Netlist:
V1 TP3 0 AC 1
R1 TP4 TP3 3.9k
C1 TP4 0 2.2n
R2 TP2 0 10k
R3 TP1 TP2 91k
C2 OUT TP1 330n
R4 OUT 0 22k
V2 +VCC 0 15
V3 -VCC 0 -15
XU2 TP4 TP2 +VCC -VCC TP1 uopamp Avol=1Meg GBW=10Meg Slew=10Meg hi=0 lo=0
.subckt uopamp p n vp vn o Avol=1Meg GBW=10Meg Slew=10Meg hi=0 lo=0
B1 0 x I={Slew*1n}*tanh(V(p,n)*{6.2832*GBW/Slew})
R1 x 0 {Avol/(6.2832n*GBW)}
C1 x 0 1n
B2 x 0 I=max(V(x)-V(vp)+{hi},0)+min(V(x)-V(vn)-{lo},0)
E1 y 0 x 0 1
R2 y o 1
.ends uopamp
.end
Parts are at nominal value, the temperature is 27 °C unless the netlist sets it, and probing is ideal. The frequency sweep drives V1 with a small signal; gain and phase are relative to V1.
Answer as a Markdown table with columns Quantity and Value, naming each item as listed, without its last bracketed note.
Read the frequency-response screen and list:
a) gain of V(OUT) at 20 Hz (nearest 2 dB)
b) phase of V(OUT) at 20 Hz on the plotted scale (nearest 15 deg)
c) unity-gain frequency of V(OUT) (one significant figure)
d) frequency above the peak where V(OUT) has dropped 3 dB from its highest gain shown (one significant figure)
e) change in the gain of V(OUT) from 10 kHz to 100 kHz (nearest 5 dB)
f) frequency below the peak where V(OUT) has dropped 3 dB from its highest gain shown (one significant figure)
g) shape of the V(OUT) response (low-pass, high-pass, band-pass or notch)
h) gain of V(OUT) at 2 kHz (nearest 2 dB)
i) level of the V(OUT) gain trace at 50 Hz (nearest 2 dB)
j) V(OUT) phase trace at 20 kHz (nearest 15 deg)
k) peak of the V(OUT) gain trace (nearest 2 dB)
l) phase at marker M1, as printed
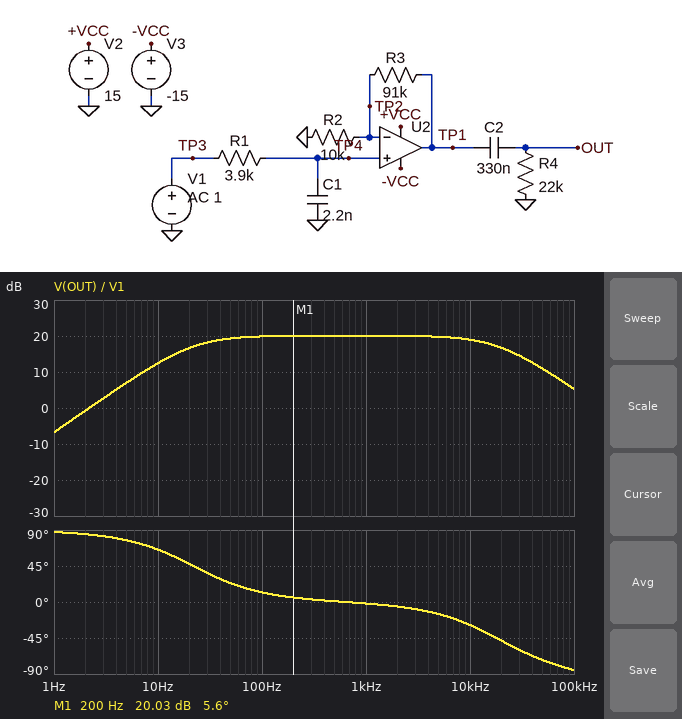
| Quantity | Value |
|---|---|
| gain of V(OUT) at 20 Hz | 16 dB |
| phase of V(OUT) at 20 Hz on the plotted scale | 45 deg |
| unity-gain frequency of V(OUT) | 2 Hz |
| frequency above the peak where V(OUT) has dropped 3 dB from its highest gain shown | 20 kHz |
| change in the gain of V(OUT) from 10 kHz to 100 kHz | -15 dB |
| frequency below the peak where V(OUT) has dropped 3 dB from its highest gain shown | 20 Hz |
| shape of the V(OUT) response | band-pass |
| gain of V(OUT) at 2 kHz | 20 dB |
| level of the V(OUT) gain trace at 50 Hz | 20 dB |
| V(OUT) phase trace at 20 kHz | -45 deg |
| peak of the V(OUT) gain trace | 20 dB |
| phase at marker M1, as printed | 5.6 deg |
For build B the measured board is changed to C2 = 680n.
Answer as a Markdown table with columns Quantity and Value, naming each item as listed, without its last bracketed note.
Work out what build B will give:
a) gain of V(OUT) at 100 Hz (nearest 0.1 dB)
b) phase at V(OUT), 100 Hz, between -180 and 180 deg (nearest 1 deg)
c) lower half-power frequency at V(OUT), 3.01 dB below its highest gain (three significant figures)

| Quantity | Value |
|---|---|
| gain of V(OUT) at 100 Hz | 20.0 dB |
| phase at V(OUT), 100 Hz, between -180 and 180 deg | 6 deg |
| lower half-power frequency at V(OUT), 3.01 dB below its highest gain | 10.6 Hz |
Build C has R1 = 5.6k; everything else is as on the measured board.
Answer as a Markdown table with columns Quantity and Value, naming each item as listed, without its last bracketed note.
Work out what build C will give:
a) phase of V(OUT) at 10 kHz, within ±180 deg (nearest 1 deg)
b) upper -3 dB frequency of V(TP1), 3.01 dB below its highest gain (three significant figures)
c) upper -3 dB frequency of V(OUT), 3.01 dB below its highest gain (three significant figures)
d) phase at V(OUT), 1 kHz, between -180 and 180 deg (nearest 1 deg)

| Quantity | Value |
|---|---|
| phase of V(OUT) at 10 kHz, within ±180 deg | -38 deg |
| upper -3 dB frequency of V(TP1), 3.01 dB below its highest gain | 12.9 kHz |
| upper -3 dB frequency of V(OUT), 3.01 dB below its highest gain | 13.0 kHz |
| phase at V(OUT), 1 kHz, between -180 and 180 deg | -3 deg |
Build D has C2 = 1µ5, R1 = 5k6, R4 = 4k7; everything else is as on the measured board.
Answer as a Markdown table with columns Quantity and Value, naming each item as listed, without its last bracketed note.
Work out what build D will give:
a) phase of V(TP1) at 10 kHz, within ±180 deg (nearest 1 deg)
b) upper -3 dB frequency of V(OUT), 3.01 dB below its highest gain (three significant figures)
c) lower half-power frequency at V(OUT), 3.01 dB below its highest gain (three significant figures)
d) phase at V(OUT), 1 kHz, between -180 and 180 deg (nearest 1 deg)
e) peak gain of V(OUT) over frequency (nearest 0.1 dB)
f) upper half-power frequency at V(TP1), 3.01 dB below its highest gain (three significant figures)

| Quantity | Value |
|---|---|
| phase of V(TP1) at 10 kHz, within ±180 deg | -38 deg |
| upper -3 dB frequency of V(OUT), 3.01 dB below its highest gain | 13.0 kHz |
| lower half-power frequency at V(OUT), 3.01 dB below its highest gain | 22.5 Hz |
| phase at V(OUT), 1 kHz, between -180 and 180 deg | -3 deg |
| peak gain of V(OUT) over frequency | 20.1 dB |
| upper half-power frequency at V(TP1), 3.01 dB below its highest gain | 12.9 kHz |
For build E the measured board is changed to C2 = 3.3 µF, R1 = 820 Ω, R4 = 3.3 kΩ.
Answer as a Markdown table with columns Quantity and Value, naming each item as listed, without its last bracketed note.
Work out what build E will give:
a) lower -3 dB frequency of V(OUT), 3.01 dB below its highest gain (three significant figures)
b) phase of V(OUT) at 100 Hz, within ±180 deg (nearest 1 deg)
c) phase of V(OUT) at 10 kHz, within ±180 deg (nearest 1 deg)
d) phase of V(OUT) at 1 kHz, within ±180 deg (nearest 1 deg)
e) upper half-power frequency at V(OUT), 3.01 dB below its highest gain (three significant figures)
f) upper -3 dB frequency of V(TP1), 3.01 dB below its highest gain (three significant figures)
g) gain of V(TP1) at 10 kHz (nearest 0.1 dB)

| Quantity | Value |
|---|---|
| lower -3 dB frequency of V(OUT), 3.01 dB below its highest gain | 14.6 Hz |
| phase of V(OUT) at 100 Hz, within ±180 deg | 8 deg |
| phase of V(OUT) at 10 kHz, within ±180 deg | -7 deg |
| phase of V(OUT) at 1 kHz, within ±180 deg | 0 deg |
| upper half-power frequency at V(OUT), 3.01 dB below its highest gain | 87.6 kHz |
| upper -3 dB frequency of V(TP1), 3.01 dB below its highest gain | 87.5 kHz |
| gain of V(TP1) at 10 kHz | 20.0 dB |
